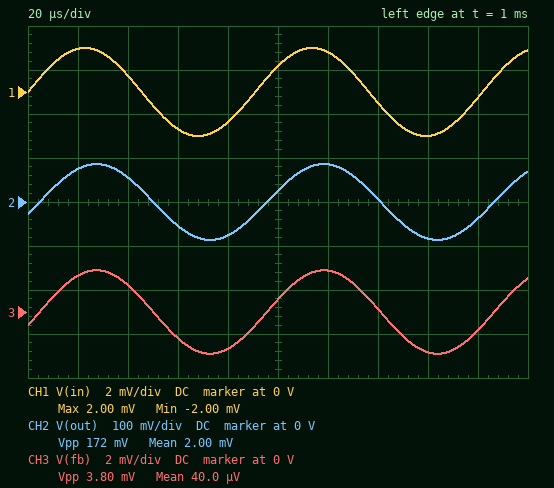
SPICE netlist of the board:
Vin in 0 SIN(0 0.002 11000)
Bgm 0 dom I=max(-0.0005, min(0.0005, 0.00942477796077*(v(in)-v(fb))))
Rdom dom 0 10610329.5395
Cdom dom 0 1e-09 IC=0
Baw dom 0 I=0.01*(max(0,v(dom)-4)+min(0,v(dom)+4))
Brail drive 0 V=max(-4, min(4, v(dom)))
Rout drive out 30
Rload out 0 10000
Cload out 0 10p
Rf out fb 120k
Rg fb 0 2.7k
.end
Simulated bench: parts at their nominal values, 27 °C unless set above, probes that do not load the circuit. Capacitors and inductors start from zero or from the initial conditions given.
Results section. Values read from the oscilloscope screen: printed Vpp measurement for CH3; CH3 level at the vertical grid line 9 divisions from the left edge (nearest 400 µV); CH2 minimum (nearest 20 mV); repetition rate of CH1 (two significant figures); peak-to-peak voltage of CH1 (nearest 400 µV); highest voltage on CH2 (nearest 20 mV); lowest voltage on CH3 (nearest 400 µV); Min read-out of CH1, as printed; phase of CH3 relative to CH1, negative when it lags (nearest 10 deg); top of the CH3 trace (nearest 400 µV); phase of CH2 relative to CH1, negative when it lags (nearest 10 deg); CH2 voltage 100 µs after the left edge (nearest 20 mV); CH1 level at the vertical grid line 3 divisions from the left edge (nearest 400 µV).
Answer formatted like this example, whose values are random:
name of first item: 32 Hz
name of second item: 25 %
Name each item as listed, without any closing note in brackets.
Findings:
printed Vpp measurement for CH3: 3.80 mV
CH3 level at the vertical grid line 9 divisions from the left edge: -800 µV
CH2 minimum: -80 mV
repetition rate of CH1: 11 kHz
peak-to-peak voltage of CH1: 4.0 mV
highest voltage on CH2: 80 mV
lowest voltage on CH3: -2.0 mV
Min read-out of CH1, as printed: -2.00 mV
phase of CH3 relative to CH1, negative when it lags: -20 deg
top of the CH3 trace: 2.0 mV
phase of CH2 relative to CH1, negative when it lags: -20 deg
CH2 voltage 100 µs after the left edge: 20 mV
CH1 level at the vertical grid line 3 divisions from the left edge: -1.6 mV
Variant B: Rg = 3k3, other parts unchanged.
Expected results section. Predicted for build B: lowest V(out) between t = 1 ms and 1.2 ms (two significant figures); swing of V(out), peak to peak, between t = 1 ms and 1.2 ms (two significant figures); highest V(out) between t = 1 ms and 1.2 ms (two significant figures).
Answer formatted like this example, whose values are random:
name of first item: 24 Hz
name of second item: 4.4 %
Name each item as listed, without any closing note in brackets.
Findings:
lowest V(out) between t = 1 ms and 1.2 ms: -72 mV
swing of V(out), peak to peak, between t = 1 ms and 1.2 ms: 140 mV
highest V(out) between t = 1 ms and 1.2 ms: 72 mV
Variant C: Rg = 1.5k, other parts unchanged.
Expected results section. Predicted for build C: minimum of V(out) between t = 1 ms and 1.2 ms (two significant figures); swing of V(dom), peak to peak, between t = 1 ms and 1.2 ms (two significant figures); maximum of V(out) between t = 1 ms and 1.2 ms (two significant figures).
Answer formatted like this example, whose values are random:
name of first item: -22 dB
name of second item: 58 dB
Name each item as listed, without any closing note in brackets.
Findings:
minimum of V(out) between t = 1 ms and 1.2 ms: -140 mV
swing of V(dom), peak to peak, between t = 1 ms and 1.2 ms: 280 mV
maximum of V(out) between t = 1 ms and 1.2 ms: 140 mV
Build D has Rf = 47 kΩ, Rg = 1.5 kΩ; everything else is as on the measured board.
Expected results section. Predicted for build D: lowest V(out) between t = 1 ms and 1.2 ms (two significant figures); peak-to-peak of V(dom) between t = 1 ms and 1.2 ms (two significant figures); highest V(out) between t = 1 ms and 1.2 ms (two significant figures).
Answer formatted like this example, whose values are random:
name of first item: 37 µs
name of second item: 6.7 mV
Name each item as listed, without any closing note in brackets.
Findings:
lowest V(out) between t = 1 ms and 1.2 ms: -63 mV
peak-to-peak of V(dom) between t = 1 ms and 1.2 ms: 130 mV
highest V(out) between t = 1 ms and 1.2 ms: 63 mV
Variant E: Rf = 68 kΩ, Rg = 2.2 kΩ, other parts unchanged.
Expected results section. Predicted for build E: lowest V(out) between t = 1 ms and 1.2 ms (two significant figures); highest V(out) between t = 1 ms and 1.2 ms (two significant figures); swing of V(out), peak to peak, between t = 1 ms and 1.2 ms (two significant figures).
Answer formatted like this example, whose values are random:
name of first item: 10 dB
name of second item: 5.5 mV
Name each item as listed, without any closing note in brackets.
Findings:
lowest V(out) between t = 1 ms and 1.2 ms: -62 mV
highest V(out) between t = 1 ms and 1.2 ms: 62 mV
swing of V(out), peak to peak, between t = 1 ms and 1.2 ms: 120 mV
